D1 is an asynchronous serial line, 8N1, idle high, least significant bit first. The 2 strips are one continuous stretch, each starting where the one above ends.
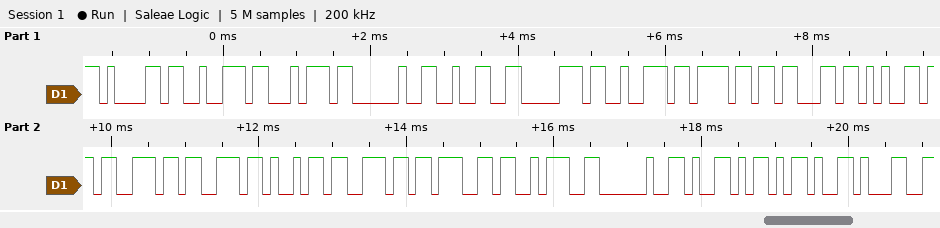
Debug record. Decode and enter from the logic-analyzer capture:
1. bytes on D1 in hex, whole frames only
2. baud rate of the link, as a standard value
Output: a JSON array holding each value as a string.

["0x61 0x72 0x74 0x20 0x32 0x70 0x72 0x6F 0x63 0x65 0x73 0x73 0x69 0x6E 0x67 0x3A 0x20 0x59 0x2D 0x31", "9600 baud"]
